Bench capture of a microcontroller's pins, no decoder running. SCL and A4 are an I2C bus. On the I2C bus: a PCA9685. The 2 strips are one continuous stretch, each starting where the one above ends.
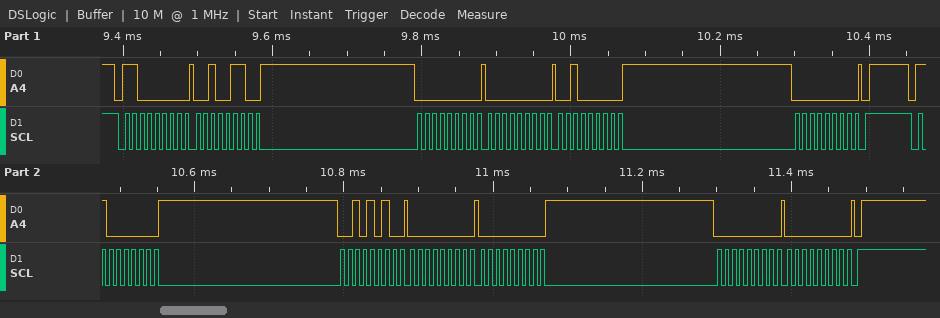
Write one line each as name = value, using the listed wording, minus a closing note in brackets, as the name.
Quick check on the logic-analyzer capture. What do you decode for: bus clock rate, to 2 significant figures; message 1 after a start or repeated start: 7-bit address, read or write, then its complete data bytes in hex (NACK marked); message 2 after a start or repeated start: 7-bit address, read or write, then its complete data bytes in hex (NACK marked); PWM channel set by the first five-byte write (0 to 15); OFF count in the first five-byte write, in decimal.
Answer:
bus clock rate, to 2 significant figures = 100 kHz
message 1 after a start or repeated start: 7-bit address, read or write, then its complete data bytes in hex = 0x60 write: 26 00 00 20 00
message 2 after a start or repeated start: 7-bit address, read or write, then its complete data bytes in hex = 0x60 write: 2A 00 00 00 00
PWM channel set by the first five-byte write = 8
OFF count in the first five-byte write, in decimal = 32
